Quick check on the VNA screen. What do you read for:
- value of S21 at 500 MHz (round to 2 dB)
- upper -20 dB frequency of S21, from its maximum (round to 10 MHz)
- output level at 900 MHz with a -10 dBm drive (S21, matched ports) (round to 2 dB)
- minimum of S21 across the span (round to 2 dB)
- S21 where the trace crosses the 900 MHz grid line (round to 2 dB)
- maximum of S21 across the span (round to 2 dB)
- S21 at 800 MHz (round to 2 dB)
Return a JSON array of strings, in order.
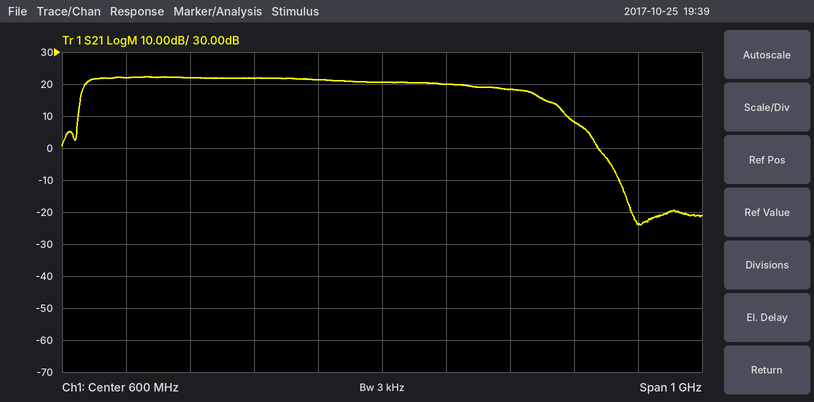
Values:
["22 dB", "930 MHz", "-2 dBm", "-24 dB", "8 dB", "22 dB", "18 dB"]
